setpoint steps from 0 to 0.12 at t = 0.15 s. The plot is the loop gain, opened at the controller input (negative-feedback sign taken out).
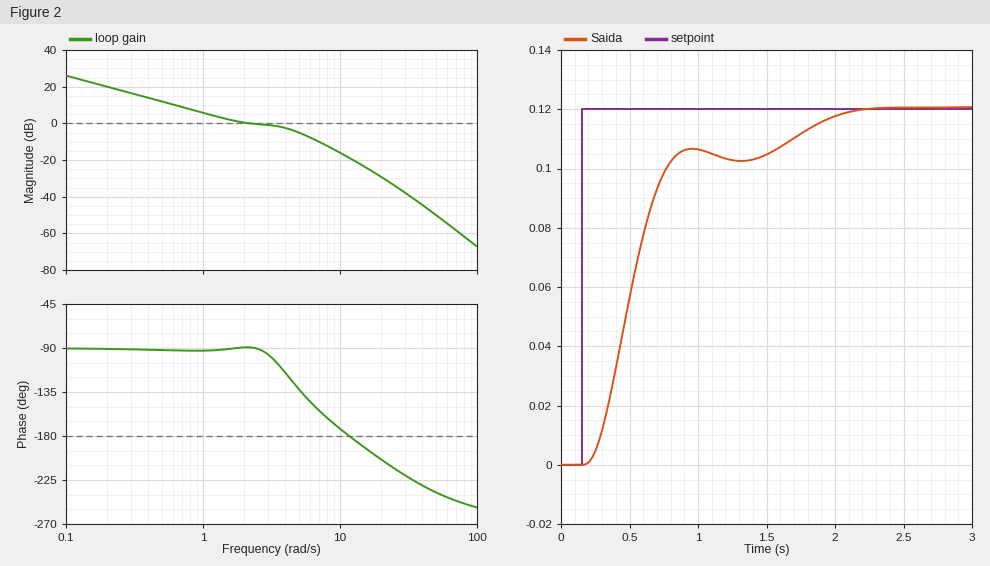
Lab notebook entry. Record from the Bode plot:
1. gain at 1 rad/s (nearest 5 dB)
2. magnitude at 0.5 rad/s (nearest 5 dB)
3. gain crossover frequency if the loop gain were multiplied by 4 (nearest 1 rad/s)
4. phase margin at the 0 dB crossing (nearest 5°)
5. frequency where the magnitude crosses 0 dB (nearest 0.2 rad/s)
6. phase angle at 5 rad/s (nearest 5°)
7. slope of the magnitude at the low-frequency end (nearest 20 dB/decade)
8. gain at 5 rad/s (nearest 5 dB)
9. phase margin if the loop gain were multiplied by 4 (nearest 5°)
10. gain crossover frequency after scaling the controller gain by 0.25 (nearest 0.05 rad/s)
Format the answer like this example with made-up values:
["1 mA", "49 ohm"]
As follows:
["5 dB", "10 dB", "8 rad/s", "90°", "2.2 rad/s", "-130°", "-20 dB/decade", "-5 dB", "20°", "0.50 rad/s"]
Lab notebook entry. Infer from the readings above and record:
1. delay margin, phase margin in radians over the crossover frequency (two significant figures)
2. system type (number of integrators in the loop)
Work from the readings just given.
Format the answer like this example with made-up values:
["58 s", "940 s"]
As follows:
["0.71 s", "1"]
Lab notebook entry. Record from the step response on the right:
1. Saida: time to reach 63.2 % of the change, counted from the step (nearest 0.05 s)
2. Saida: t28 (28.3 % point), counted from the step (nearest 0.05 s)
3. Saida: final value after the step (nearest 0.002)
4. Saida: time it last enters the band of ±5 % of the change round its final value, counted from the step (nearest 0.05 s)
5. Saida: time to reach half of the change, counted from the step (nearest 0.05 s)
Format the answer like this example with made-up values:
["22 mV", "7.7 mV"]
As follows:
["0.45 s", "0.25 s", "0.120", "1.70 s", "0.35 s"]
